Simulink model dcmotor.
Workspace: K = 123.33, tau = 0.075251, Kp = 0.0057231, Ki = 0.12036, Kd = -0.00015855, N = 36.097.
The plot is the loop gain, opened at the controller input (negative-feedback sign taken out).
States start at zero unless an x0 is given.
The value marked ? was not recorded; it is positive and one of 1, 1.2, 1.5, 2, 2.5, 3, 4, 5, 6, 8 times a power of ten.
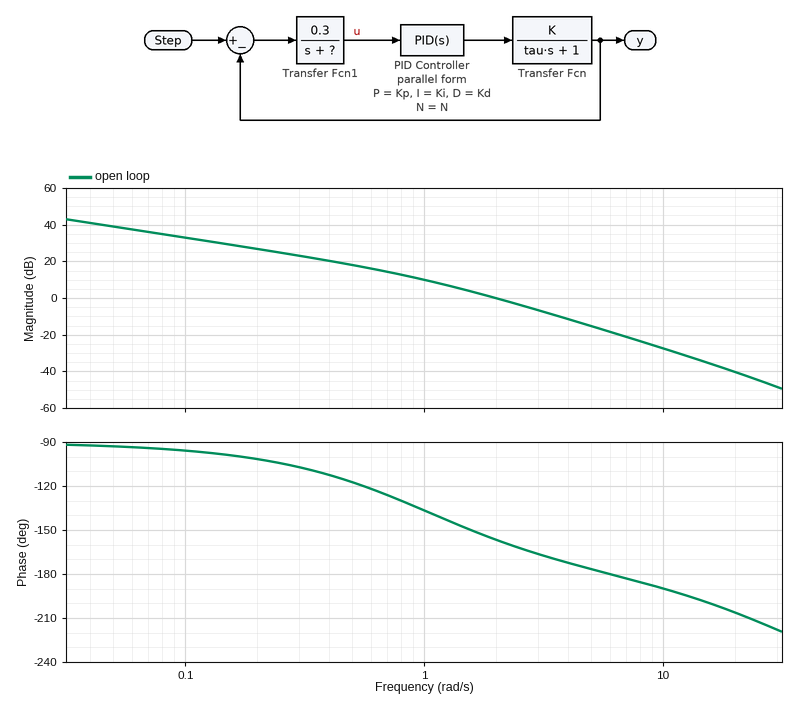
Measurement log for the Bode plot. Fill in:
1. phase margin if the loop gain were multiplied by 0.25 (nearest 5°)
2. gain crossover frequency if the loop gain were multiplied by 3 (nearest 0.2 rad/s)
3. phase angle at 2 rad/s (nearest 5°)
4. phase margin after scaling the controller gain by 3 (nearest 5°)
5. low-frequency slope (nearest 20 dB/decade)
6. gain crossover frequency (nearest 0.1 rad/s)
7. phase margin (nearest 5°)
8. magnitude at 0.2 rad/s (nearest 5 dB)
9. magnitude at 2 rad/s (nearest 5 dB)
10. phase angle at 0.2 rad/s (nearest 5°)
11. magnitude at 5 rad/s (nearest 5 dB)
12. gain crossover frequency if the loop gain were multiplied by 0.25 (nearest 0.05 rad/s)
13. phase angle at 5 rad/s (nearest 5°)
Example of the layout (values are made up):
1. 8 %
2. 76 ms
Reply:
1. 50°
2. 3.6 rad/s
3. -155°
4. 10°
5. -20 dB/decade
6. 2.0 rad/s
7. 25°
8. 25 dB
9. 0 dB
10. -100°
11. -15 dB
12. 0.85 rad/s
13. -175°
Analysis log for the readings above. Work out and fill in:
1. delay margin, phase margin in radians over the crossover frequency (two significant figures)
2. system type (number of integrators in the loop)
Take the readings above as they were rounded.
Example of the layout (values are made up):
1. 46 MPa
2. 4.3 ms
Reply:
1. 0.22 s
2. 1
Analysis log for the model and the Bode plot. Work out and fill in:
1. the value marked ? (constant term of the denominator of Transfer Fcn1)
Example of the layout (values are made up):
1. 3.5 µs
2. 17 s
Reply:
1. 1
